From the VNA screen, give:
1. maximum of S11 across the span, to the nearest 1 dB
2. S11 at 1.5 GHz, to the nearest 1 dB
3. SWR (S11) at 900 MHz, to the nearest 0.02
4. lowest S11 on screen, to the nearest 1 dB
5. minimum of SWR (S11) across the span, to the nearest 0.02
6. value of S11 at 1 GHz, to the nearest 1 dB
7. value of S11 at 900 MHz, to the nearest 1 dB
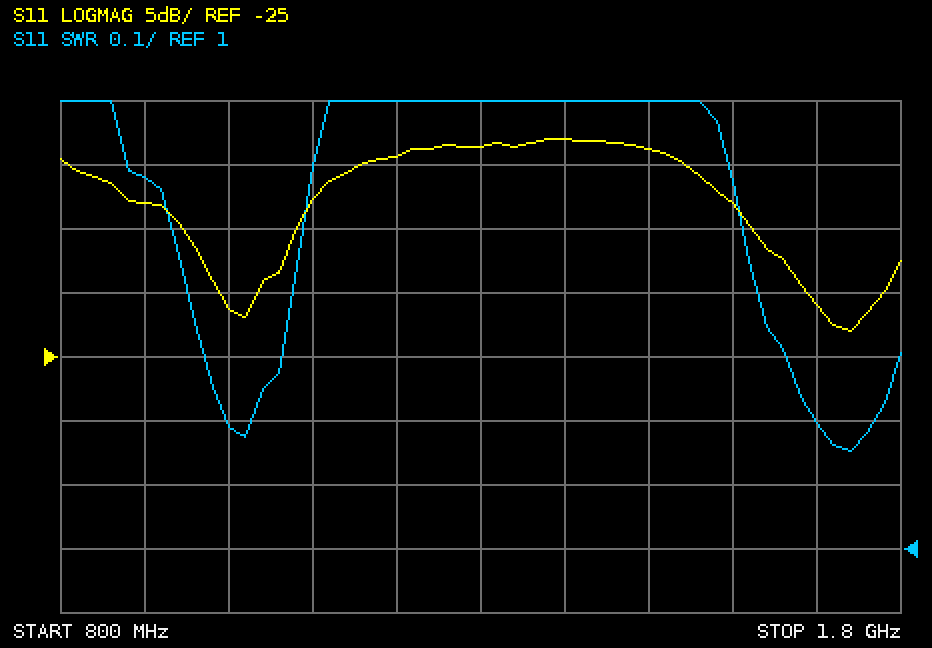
-8 dB
-9 dB
1.58
-23 dB
1.16
-21 dB
-13 dB
